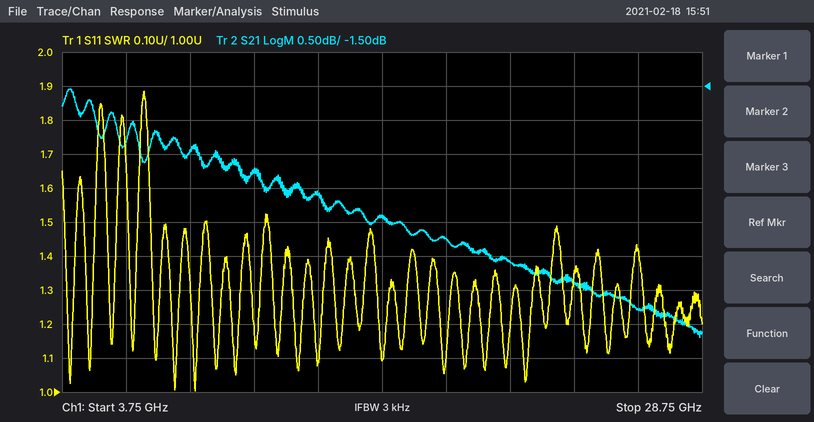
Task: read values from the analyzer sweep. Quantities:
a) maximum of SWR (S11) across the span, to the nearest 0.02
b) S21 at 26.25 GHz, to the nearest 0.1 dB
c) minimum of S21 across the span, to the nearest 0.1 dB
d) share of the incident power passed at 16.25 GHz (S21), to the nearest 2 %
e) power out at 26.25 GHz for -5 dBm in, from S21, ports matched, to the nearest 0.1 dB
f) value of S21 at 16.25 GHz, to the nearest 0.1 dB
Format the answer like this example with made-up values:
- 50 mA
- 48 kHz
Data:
- 1.88
- -4.8 dB
- -5.2 dB
- 46 %
- -9.8 dBm
- -3.4 dB
